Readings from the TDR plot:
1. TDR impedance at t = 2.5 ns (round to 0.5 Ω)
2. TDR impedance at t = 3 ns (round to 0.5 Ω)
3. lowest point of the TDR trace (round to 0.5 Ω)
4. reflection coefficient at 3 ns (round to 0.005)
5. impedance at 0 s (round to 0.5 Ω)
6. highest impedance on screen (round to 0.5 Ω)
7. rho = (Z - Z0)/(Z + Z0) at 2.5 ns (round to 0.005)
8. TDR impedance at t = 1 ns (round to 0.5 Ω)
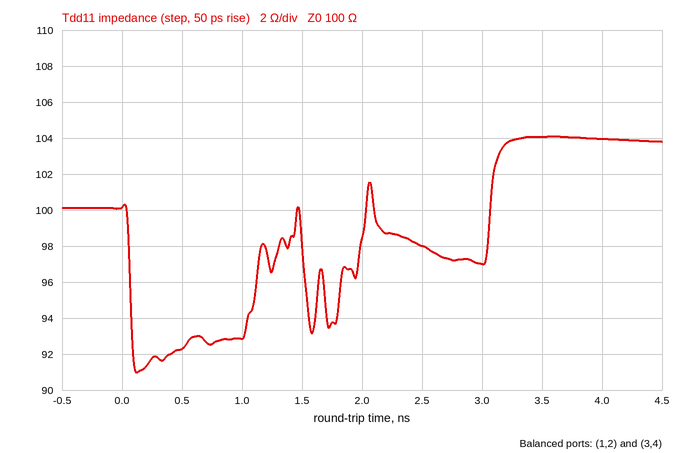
98.0 Ω
97.0 Ω
91.0 Ω
-0.015
100.0 Ω
104.0 Ω
-0.010
93.0 Ω
